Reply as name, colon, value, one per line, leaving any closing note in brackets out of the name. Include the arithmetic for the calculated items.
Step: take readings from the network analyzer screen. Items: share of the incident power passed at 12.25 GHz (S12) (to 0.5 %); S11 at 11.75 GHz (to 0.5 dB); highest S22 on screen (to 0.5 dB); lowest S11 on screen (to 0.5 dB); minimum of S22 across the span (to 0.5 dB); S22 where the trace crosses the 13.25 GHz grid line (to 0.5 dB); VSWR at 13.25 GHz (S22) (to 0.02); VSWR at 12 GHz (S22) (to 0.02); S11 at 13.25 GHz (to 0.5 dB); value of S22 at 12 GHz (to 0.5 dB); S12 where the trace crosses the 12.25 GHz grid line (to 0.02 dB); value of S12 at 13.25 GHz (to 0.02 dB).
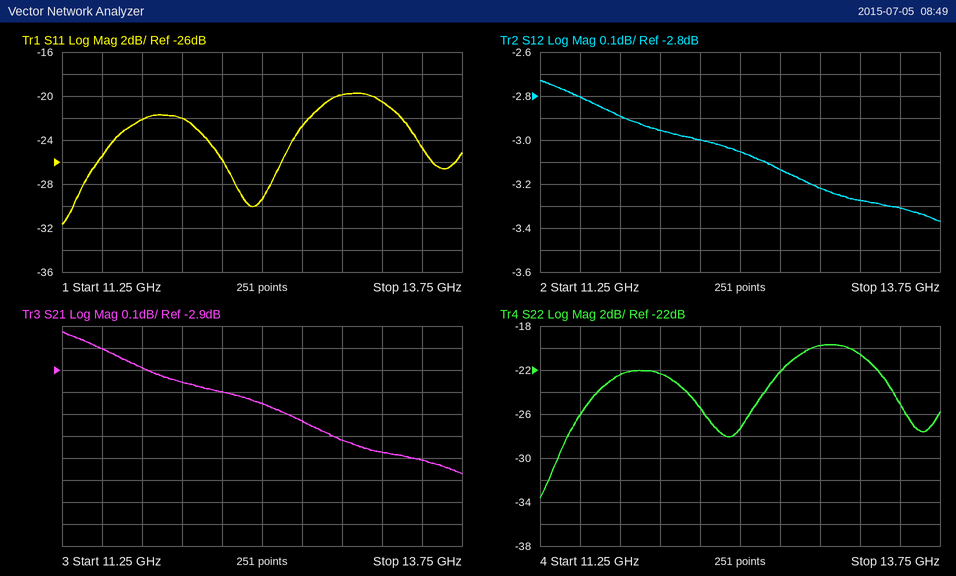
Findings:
share of the incident power passed at 12.25 GHz (S12): 10^(-3/10) ≈ 50.1 %, so 50.0 % to the nearest 0.5 %
S11 at 11.75 GHz: -22.0 dB
highest S22 on screen: -19.5 dB
lowest S11 on screen: -31.5 dB
minimum of S22 across the span: -33.5 dB
S22 where the trace crosses the 13.25 GHz grid line: -20.5 dB
VSWR at 13.25 GHz (S22): |Γ| = 10^(-20.5/20) = 0.0944; VSWR = (1 + 0.0944)/(1 − 0.0944) ≈ 1.21, so 1.20 to the nearest 0.02
VSWR at 12 GHz (S22): |Γ| = 10^(-22.5/20) = 0.0750; VSWR = (1 + 0.0750)/(1 − 0.0750) ≈ 1.16
S11 at 13.25 GHz: -20.5 dB
value of S22 at 12 GHz: -22.5 dB
S12 where the trace crosses the 12.25 GHz grid line: -3.00 dB
value of S12 at 13.25 GHz: -3.28 dB
